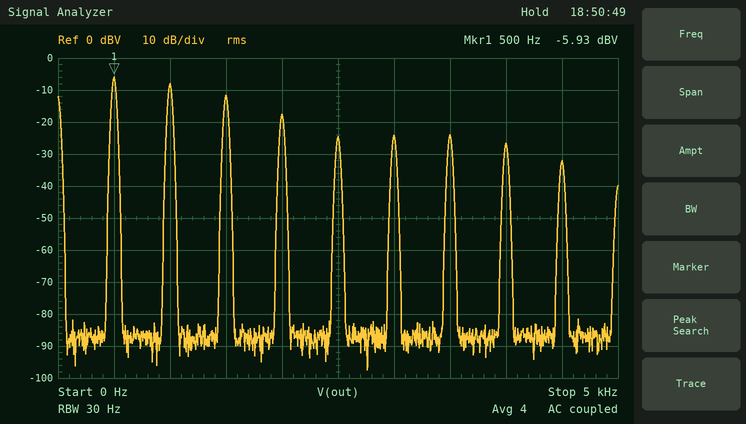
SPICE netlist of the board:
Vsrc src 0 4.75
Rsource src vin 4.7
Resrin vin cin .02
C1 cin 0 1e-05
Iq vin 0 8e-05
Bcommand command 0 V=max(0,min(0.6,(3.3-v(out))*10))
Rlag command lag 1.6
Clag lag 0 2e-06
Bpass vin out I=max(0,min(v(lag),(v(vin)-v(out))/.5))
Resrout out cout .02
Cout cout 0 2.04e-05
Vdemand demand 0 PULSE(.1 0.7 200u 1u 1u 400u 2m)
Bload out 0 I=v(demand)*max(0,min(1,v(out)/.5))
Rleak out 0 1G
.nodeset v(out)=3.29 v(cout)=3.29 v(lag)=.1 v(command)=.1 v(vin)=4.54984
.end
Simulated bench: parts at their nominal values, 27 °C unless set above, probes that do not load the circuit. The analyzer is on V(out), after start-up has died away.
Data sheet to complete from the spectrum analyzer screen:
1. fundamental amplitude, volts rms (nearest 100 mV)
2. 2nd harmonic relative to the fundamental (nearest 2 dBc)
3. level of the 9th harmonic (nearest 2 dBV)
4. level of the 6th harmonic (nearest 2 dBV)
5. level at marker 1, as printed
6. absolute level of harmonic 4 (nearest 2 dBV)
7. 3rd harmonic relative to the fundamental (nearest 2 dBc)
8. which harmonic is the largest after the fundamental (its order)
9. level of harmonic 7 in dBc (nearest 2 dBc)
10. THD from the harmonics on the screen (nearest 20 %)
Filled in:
500 mV
-2 dBc
-32 dBV
-24 dBV
-5.93 dBV
-18 dBV
-6 dBc
2
-18 dBc
100 %
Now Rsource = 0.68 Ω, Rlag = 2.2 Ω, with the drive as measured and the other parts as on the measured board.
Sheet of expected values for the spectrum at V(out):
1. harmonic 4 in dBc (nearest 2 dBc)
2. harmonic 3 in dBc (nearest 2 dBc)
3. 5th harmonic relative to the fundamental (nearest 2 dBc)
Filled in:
-8 dBc
-4 dBc
-12 dBc
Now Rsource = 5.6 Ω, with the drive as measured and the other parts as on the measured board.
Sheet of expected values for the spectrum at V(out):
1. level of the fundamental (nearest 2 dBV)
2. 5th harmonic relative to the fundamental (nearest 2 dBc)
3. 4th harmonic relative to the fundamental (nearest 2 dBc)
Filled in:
-4 dBV
-24 dBc
-14 dBc
